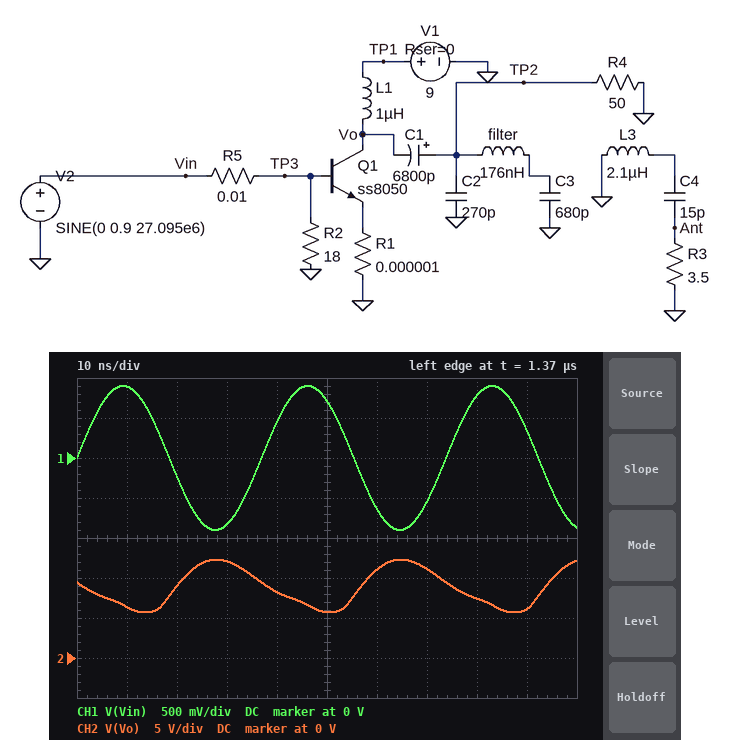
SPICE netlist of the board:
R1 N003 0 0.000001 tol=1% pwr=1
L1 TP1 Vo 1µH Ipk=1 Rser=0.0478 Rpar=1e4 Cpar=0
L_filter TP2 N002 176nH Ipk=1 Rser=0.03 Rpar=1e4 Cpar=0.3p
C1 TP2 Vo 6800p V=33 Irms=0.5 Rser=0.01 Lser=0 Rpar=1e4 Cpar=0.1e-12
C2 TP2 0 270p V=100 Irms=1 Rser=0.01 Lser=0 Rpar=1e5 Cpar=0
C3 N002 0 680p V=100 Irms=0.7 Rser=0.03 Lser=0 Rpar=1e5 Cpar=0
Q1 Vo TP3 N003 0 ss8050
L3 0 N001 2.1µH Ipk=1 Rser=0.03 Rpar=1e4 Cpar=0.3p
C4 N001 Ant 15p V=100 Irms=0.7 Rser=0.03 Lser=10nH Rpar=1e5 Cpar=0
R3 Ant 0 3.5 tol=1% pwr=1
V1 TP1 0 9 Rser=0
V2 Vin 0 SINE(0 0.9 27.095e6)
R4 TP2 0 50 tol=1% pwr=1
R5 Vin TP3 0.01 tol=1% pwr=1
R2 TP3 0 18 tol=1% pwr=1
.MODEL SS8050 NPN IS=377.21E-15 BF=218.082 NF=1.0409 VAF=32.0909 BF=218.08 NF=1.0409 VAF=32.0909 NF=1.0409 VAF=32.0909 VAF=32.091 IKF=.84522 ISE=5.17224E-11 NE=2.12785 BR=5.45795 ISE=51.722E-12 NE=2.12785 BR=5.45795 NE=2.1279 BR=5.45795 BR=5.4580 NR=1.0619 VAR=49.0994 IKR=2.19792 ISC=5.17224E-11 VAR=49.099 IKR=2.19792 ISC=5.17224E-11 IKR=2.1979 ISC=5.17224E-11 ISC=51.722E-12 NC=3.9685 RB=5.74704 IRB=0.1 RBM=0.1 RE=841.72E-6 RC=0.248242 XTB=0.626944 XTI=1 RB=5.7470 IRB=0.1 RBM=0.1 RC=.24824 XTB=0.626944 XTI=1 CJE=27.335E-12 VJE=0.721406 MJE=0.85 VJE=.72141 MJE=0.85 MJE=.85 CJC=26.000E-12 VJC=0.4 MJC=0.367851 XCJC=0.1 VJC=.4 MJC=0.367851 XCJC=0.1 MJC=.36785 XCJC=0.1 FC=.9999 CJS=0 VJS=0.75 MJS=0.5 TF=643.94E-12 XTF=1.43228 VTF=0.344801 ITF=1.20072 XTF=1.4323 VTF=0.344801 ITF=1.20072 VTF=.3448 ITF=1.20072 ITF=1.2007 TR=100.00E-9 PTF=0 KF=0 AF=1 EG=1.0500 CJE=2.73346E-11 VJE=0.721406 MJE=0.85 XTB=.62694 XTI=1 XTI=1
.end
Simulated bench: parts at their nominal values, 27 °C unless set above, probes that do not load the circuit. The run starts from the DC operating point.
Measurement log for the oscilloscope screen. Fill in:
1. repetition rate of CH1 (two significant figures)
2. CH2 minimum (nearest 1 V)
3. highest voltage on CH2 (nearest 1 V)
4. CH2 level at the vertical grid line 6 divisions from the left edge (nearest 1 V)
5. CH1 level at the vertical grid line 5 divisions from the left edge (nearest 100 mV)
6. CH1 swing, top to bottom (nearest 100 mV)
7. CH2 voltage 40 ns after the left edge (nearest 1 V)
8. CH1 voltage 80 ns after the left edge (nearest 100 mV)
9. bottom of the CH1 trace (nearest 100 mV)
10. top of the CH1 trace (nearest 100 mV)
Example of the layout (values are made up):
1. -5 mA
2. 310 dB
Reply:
1. 27 MHz
2. 6 V
3. 12 V
4. 11 V
5. 700 mV
6. 1.8 V
7. 8 V
8. 800 mV
9. -900 mV
10. 900 mV
